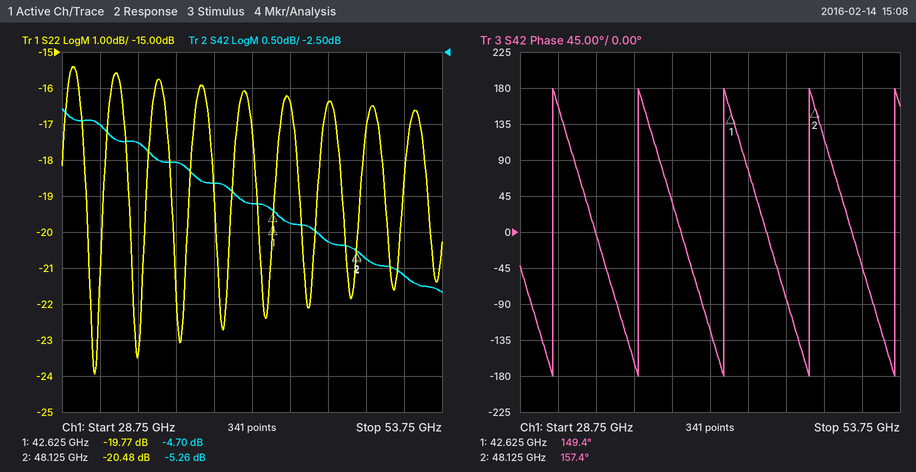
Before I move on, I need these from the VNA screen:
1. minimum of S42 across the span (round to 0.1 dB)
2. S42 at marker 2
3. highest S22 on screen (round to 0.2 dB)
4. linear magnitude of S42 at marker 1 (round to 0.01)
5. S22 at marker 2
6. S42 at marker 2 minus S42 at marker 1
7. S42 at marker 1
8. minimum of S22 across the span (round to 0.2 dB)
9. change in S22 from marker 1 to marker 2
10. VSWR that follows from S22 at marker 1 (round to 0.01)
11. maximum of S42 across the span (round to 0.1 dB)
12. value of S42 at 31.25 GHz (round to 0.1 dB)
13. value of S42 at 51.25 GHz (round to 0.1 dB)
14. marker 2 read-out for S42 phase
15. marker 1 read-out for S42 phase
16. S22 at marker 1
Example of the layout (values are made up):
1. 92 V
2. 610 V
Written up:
1. -5.8 dB
2. -5.26 dB
3. -15.4 dB
4. 0.58
5. -20.48 dB
6. -0.56 dB
7. -4.70 dB
8. -24.0 dB
9. -0.71 dB
10. 1.23
11. -3.3 dB
12. -3.5 dB
13. -5.6 dB
14. 157.4°
15. 149.4°
16. -19.77 dB
